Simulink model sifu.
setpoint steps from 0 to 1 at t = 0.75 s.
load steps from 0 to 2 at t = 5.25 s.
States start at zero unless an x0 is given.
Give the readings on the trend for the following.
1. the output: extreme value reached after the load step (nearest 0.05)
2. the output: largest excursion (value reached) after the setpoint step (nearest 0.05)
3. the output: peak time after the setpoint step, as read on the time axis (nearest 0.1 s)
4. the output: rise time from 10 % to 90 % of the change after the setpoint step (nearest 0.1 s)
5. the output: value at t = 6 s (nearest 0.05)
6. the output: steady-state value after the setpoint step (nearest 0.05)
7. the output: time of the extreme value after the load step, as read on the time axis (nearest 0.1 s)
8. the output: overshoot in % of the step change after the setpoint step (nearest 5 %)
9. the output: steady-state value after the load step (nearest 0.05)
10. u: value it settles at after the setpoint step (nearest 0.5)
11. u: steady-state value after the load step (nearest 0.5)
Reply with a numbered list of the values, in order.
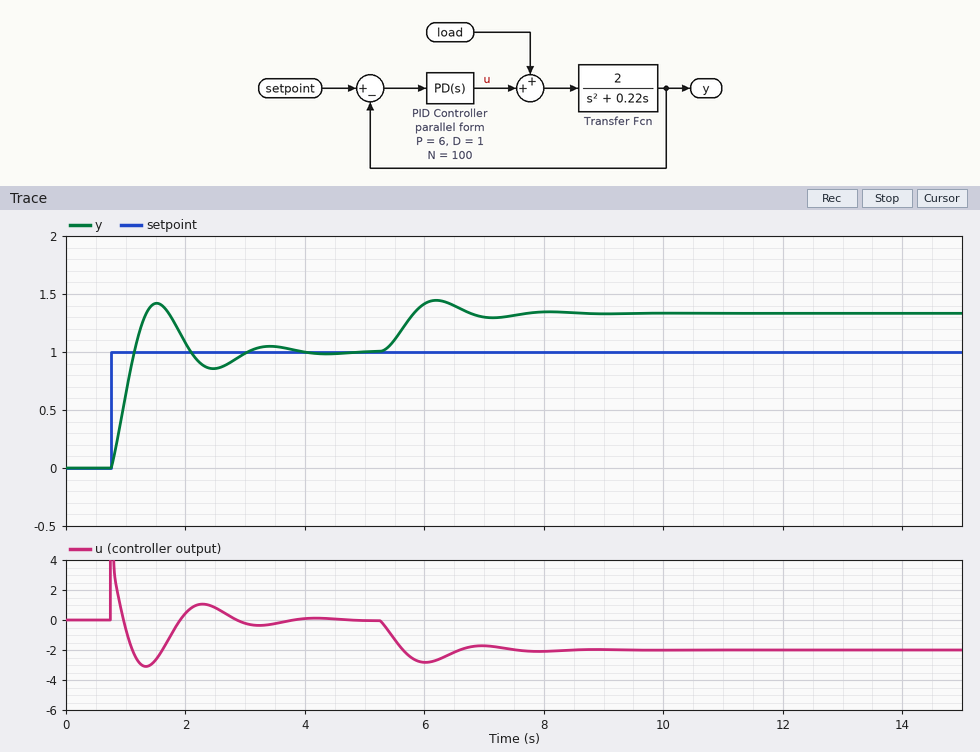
1. 1.45
2. 1.40
3. 1.5 s
4. 0.3 s
5. 1.40
6. 1.00
7. 6.2 s
8. 40 %
9. 1.35
10. 0.0
11. -2.0
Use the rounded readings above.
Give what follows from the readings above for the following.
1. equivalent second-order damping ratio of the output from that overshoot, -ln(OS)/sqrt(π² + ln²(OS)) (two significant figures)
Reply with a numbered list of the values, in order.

1. 0.28
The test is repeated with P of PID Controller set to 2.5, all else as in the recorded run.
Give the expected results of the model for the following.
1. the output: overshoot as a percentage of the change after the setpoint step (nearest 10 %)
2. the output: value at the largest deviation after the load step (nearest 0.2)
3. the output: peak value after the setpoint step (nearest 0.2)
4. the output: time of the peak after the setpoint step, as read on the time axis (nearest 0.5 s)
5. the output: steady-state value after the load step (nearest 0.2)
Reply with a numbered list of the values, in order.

1. 30 %
2. 2.0
3. 1.2
4. 2.0 s
5. 1.8
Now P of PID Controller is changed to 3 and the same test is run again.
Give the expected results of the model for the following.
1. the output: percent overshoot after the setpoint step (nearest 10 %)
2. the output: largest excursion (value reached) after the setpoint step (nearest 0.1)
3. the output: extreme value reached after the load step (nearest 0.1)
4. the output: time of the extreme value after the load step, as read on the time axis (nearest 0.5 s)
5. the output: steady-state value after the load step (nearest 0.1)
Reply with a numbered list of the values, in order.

1. 30 %
2. 1.3
3. 1.8
4. 6.5 s
5. 1.7
